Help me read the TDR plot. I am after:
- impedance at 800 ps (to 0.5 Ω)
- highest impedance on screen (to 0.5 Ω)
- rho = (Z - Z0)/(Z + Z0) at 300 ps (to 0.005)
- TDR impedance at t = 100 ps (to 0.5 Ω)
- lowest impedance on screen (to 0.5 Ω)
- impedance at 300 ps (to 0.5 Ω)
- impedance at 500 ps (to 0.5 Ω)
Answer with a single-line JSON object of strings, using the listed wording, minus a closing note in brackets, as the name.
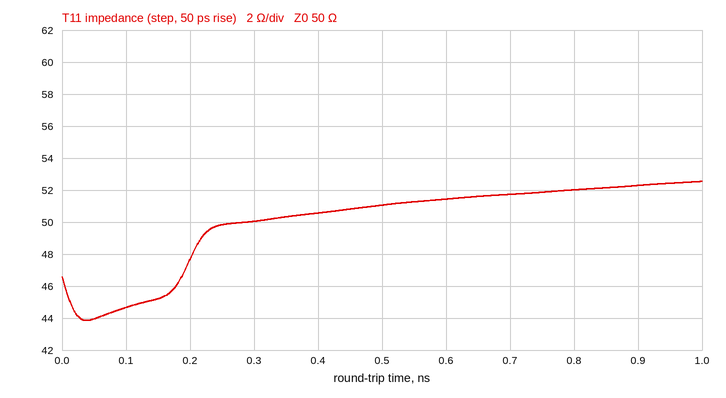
{"impedance at 800 ps": "52.0 Ω", "highest impedance on screen": "52.5 Ω", "rho = (Z - Z0)/(Z + Z0) at 300 ps": "0.000", "TDR impedance at t = 100 ps": "44.5 Ω", "lowest impedance on screen": "44.0 Ω", "impedance at 300 ps": "50.0 Ω", "impedance at 500 ps": "51.0 Ω"}
